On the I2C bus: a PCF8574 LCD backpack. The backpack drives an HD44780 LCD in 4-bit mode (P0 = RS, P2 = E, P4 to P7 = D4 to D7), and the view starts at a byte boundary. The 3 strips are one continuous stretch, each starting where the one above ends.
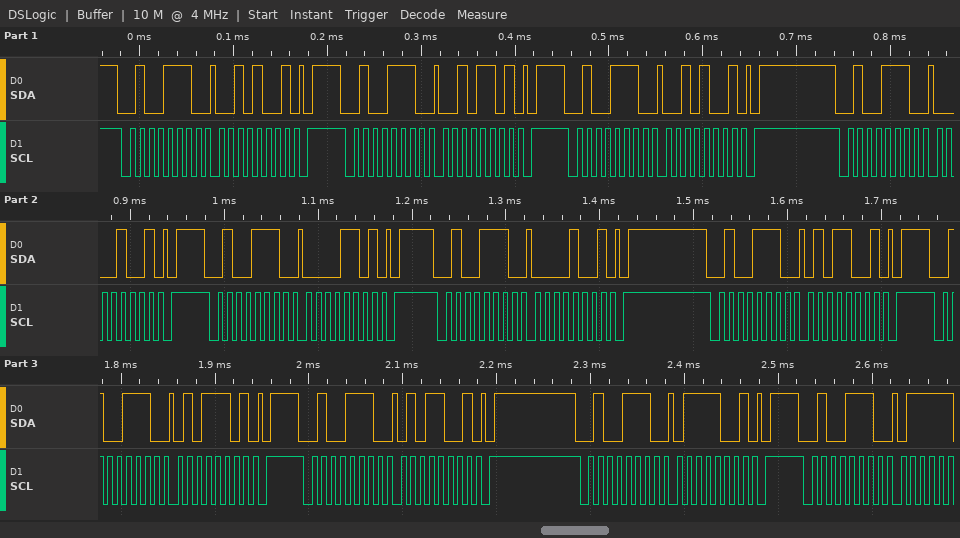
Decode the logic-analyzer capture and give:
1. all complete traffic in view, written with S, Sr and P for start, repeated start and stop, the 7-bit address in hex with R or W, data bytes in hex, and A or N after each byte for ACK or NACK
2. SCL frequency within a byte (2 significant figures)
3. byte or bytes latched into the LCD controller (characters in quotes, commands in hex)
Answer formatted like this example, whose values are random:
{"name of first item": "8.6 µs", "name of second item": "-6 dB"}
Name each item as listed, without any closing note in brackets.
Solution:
{"all complete traffic in view, written with S, Sr and P for start, repeated start and stop, the 7-bit address in hex with R or W, data bytes in hex, and A or N after each byte for ACK or NACK": "S 27W A 29 A P S 27W A 2D A P S 27W A 29 A P S 27W A 09 A P S 27W A 0D A P S 27W A 09 A P S 27W A 59 A P S 27W A 5D A P S 27W A 59 A P S 27W A 79 A P S 27W A", "SCL frequency within a byte": "100 kHz", "byte or bytes latched into the LCD controller": "' '"}
